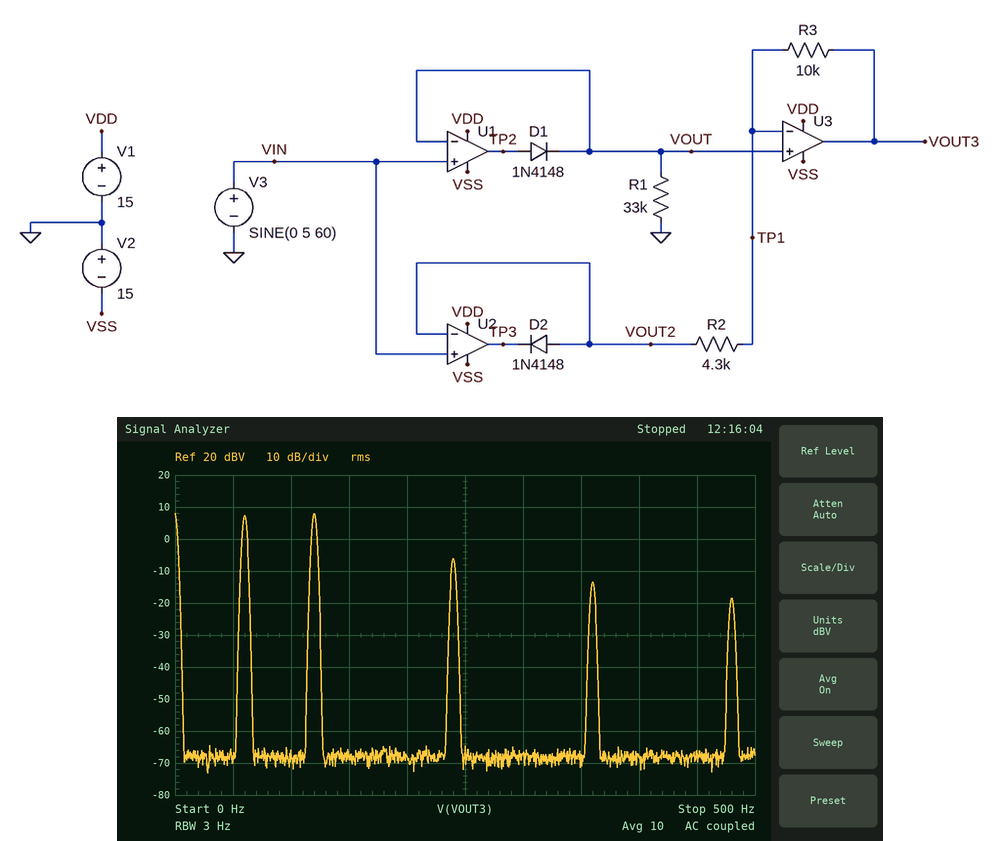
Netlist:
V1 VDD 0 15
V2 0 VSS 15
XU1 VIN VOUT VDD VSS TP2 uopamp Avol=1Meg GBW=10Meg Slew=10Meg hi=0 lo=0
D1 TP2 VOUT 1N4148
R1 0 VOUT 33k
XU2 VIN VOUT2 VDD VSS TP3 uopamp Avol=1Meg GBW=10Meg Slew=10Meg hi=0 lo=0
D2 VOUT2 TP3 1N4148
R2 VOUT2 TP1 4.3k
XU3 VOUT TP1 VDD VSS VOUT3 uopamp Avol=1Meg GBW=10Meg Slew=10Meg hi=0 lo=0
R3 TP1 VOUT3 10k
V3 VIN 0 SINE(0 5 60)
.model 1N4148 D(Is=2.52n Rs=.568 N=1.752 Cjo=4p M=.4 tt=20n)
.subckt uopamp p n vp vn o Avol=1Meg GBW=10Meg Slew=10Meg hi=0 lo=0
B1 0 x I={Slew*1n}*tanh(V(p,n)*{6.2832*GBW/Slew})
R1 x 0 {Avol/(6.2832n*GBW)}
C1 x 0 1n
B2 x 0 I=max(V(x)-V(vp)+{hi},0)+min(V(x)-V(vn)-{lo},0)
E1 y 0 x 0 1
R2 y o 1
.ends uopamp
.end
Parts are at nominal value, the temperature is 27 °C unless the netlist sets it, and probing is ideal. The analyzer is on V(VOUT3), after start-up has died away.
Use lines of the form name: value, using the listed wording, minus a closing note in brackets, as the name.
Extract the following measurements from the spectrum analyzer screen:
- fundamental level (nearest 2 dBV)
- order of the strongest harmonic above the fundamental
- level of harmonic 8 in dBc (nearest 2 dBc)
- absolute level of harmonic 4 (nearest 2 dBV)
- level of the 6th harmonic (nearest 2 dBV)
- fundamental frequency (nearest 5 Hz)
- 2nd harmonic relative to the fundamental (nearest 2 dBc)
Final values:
fundamental level: 8 dBV
order of the strongest harmonic above the fundamental: 2
level of harmonic 8 in dBc: -26 dBc
absolute level of harmonic 4: -6 dBV
level of the 6th harmonic: -14 dBV
fundamental frequency: 60 Hz
2nd harmonic relative to the fundamental: 0 dBc
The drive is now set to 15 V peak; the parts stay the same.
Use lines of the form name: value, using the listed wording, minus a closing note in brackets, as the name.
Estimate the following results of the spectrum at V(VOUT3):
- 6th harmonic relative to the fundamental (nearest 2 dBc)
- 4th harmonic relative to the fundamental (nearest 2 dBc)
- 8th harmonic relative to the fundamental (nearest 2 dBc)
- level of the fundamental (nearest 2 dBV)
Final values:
6th harmonic relative to the fundamental: -2 dBc
4th harmonic relative to the fundamental: 2 dBc
8th harmonic relative to the fundamental: -6 dBc
level of the fundamental: 2 dBV
